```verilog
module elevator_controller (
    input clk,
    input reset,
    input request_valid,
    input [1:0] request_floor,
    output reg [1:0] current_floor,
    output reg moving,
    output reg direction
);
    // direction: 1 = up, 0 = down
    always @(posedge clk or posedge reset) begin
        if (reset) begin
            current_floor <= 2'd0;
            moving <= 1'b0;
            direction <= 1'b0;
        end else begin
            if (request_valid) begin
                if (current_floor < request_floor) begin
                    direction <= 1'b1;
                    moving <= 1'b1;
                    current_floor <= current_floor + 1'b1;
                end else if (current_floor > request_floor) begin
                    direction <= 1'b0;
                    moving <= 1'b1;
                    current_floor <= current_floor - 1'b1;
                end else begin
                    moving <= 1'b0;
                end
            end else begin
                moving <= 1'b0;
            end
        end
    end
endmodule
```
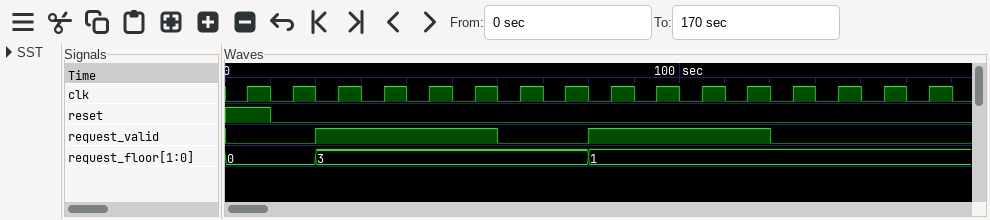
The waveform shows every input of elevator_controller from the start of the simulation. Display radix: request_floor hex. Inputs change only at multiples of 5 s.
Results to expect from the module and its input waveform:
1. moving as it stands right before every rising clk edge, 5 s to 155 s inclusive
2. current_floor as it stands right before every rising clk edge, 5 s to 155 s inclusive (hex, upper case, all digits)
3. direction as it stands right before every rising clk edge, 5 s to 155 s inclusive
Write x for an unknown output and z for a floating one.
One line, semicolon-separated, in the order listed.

0 0 0 1 1 1 0 0 0 1 1 0 0 0 0 0; 0, 0, 0, 1, 2, 3, 3, 3, 3, 2, 1, 1, 1, 1, 1, 1; 0 0 0 1 1 1 1 1 1 0 0 0 0 0 0 0
